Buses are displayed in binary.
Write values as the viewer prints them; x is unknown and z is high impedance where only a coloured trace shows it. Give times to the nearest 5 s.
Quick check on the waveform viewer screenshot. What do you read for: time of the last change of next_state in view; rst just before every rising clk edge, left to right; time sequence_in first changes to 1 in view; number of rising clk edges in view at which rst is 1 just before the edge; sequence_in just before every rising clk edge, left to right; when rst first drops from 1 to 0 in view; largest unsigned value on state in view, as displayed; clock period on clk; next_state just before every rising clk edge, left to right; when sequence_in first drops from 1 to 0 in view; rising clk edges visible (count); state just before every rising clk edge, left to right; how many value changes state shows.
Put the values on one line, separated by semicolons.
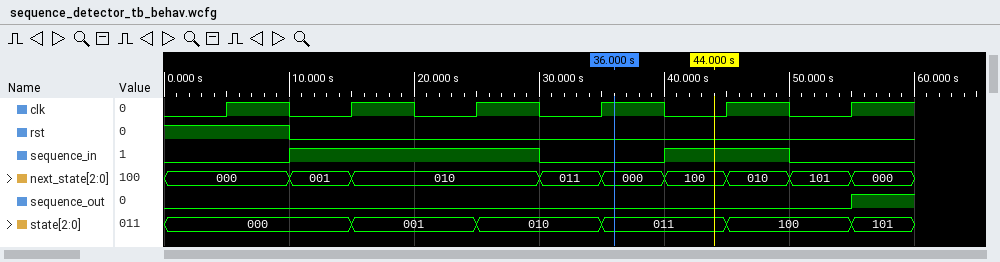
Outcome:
55 s; 1 0 0 0 0 0; 10 s; 1; 0 1 1 0 1 0; 10 s; 101; 10 s; 000, 001, 010, 011, 100, 101; 30 s; 6; 000, 000, 001, 010, 011, 100; 5
